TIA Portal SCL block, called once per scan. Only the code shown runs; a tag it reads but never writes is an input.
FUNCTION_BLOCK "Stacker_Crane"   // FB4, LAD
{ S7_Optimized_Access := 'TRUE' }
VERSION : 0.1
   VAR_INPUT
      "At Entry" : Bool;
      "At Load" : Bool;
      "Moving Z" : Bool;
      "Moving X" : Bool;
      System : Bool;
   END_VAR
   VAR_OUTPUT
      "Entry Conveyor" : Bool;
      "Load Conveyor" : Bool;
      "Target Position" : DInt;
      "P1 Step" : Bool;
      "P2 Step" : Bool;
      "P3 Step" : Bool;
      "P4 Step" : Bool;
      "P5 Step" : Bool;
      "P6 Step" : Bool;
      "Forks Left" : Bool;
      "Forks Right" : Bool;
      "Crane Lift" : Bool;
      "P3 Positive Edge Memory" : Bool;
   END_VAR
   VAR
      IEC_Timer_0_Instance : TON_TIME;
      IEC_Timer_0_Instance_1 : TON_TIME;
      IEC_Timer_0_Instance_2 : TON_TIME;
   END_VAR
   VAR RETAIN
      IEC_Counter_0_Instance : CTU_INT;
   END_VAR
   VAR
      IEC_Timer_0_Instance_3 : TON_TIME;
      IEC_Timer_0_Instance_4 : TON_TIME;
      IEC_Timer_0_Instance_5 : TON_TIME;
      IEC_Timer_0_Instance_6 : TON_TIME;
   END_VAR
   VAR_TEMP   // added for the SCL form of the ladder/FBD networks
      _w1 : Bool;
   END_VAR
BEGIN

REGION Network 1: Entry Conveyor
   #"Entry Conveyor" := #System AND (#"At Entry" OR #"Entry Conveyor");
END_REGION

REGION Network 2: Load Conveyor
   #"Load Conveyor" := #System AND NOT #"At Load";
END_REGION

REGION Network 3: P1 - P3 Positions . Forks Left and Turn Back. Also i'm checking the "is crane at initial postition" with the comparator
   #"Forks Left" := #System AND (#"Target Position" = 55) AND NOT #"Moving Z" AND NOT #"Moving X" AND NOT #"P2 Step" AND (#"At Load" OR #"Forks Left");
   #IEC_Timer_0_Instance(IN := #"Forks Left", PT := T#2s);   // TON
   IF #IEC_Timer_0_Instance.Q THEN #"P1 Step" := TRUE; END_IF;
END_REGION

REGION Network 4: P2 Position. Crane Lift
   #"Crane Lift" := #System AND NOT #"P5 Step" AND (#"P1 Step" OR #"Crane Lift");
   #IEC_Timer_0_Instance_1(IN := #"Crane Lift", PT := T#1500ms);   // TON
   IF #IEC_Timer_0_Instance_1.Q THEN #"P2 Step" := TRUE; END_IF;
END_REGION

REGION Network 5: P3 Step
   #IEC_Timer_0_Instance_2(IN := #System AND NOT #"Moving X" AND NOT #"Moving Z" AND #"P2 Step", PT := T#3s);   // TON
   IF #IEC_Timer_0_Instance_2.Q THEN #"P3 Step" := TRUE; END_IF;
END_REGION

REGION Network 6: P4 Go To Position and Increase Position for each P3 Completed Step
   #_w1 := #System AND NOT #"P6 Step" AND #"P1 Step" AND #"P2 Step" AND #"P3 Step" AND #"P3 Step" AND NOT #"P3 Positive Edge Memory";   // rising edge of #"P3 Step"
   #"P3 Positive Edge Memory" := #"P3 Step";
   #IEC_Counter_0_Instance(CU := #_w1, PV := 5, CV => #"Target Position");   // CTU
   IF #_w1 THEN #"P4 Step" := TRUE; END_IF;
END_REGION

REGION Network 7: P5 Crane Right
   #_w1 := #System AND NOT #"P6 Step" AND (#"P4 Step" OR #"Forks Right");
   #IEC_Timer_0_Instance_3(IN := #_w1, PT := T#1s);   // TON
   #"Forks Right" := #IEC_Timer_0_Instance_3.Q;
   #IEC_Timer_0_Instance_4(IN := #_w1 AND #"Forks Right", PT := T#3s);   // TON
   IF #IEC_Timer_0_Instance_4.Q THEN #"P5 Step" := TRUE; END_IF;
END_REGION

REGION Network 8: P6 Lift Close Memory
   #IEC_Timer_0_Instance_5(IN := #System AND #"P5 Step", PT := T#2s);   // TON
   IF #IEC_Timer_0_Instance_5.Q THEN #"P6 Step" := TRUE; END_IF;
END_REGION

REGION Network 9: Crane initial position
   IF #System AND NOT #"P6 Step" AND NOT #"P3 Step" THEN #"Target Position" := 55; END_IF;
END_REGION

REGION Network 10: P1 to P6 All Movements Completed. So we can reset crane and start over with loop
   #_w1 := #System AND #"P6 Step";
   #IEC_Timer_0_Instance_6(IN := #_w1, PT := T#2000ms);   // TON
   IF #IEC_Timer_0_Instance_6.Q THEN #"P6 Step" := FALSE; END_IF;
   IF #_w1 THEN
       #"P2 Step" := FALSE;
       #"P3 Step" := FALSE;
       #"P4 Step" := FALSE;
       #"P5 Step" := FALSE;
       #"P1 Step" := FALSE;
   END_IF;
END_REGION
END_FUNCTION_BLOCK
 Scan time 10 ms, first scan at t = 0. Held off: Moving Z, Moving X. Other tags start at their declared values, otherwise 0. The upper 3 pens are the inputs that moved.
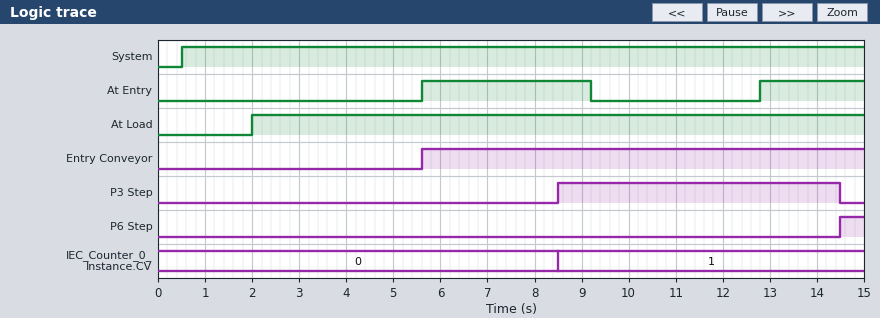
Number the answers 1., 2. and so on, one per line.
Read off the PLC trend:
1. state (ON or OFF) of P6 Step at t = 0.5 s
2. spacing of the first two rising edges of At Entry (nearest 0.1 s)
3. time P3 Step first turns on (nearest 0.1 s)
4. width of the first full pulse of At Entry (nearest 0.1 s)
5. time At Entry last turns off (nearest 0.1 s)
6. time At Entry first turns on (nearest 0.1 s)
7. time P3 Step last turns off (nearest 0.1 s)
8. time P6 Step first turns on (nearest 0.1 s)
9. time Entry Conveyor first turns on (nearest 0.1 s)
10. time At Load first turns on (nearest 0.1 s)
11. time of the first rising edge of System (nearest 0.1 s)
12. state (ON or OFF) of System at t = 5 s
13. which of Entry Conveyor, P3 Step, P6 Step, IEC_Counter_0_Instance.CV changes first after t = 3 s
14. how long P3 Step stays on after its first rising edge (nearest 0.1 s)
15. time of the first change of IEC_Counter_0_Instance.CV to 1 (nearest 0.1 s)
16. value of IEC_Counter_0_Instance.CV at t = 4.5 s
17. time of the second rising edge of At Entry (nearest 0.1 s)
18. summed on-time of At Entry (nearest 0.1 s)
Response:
1. OFF
2. 7.2 s
3. 8.5 s
4. 3.6 s
5. 9.2 s
6. 5.6 s
7. 14.5 s
8. 14.5 s
9. 5.6 s
10. 2.0 s
11. 0.5 s
12. ON
13. Entry Conveyor
14. 6.0 s
15. 8.5 s
16. 0
17. 12.8 s
18. 5.8 s
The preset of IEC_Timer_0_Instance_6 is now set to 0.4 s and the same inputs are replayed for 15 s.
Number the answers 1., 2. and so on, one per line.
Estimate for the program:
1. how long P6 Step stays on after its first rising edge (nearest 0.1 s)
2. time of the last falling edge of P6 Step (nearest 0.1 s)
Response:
1. 0.4 s
2. 14.9 s
